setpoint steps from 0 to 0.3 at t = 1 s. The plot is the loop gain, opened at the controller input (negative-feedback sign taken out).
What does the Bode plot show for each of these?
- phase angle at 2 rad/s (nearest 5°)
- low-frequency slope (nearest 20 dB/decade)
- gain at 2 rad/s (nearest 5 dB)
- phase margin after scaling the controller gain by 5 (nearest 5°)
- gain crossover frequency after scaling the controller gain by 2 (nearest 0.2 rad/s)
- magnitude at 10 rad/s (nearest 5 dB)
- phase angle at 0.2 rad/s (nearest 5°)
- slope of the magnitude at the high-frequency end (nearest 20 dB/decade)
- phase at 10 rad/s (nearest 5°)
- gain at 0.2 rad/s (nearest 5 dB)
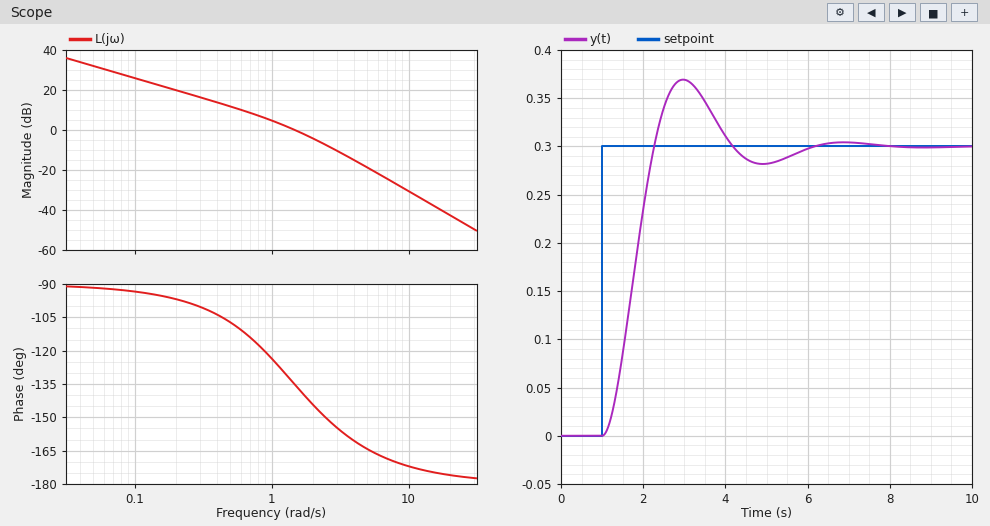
-145°
-20 dB/decade
-5 dB
20°
2.2 rad/s
-30 dB
-95°
-40 dB/decade
-170°
20 dB
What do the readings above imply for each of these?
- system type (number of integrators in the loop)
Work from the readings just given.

1
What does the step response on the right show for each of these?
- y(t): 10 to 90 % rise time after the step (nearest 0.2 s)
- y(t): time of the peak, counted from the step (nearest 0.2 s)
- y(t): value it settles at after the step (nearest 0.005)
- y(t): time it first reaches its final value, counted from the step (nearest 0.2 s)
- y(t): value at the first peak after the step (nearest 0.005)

0.8 s
2.0 s
0.300
1.2 s
0.370
